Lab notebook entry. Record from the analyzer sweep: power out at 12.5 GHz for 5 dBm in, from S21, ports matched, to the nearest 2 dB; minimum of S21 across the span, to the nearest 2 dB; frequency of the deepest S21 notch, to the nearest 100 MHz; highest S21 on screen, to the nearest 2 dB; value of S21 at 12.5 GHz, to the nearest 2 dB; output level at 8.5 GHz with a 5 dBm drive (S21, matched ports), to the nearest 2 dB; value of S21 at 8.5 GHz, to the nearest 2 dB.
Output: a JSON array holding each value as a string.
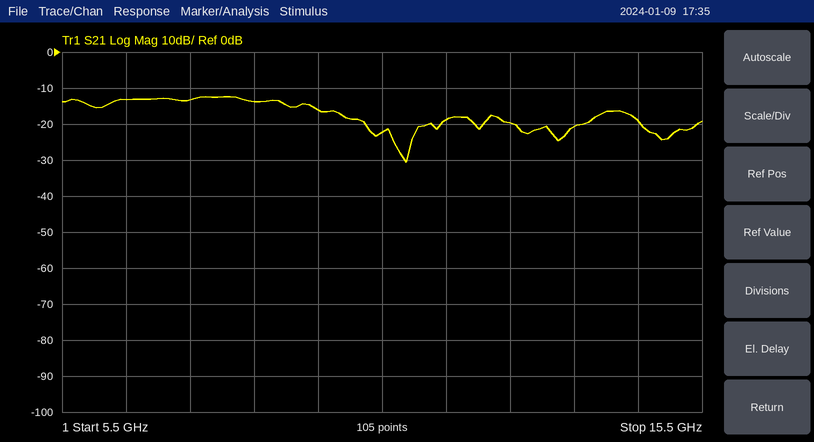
["-14 dBm", "-30 dB", "10.9 GHz", "-12 dB", "-20 dB", "-8 dBm", "-14 dB"]
